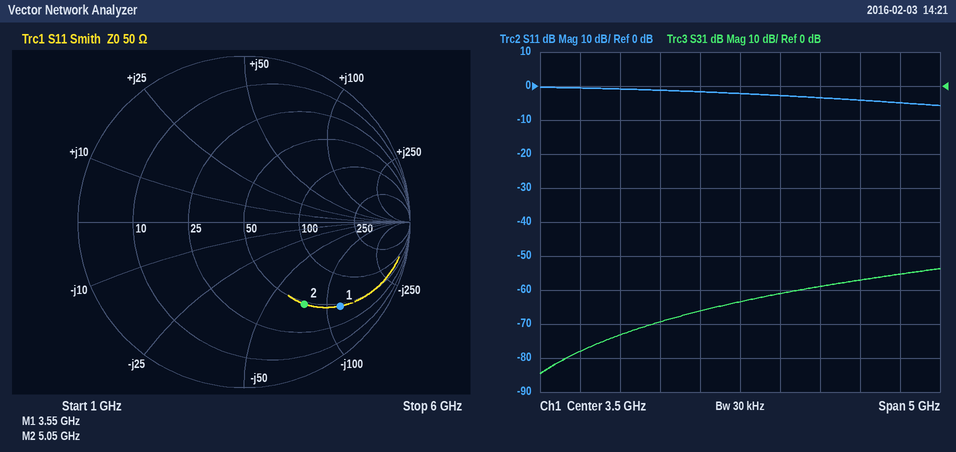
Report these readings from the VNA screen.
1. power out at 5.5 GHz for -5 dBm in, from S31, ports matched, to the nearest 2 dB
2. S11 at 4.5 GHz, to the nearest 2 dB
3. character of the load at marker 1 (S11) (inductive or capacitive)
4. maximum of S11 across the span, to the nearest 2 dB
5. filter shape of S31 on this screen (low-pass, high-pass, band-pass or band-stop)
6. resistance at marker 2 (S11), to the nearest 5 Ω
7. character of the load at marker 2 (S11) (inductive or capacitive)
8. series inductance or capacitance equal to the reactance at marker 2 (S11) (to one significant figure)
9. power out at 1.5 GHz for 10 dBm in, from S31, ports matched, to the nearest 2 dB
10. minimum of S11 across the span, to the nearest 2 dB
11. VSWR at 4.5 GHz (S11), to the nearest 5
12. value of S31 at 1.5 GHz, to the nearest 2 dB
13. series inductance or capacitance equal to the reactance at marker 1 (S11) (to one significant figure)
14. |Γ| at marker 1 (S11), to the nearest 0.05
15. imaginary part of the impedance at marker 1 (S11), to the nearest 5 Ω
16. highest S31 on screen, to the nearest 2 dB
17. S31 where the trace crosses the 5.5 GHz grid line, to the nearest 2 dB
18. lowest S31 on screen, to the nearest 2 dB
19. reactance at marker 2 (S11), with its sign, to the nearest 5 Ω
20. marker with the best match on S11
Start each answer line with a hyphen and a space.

- -60 dBm
- -4 dB
- capacitive
- 0 dB
- high-pass
- 50 Ω
- capacitive
- 400 fF
- -68 dBm
- -6 dB
- 5
- -78 dB
- 400 fF
- 0.75
- -115 Ω
- -54 dB
- -56 dB
- -84 dB
- -75 Ω
- marker 2
